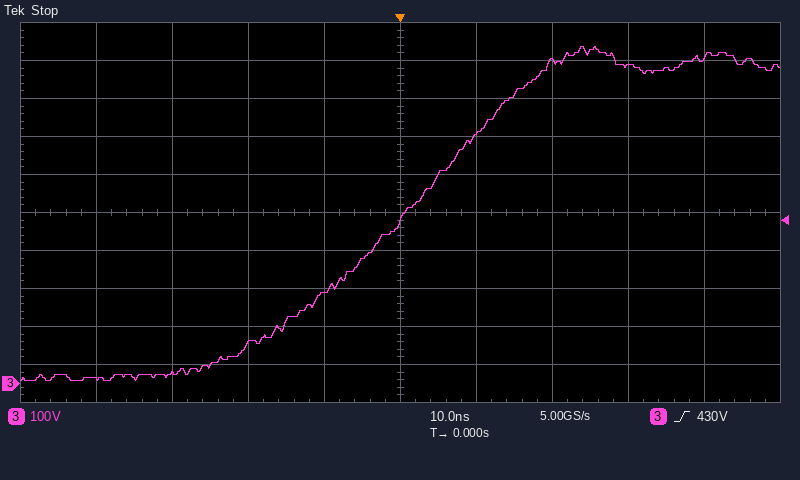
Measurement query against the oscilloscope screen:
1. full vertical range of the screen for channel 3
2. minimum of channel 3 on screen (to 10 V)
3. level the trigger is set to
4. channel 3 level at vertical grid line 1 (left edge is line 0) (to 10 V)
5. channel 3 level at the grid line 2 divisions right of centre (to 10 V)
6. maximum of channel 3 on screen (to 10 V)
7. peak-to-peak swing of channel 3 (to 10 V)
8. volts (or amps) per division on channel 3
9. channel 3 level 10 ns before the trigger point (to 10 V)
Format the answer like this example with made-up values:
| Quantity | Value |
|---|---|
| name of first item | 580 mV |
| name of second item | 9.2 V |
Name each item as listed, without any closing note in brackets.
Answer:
| Quantity | Value |
|---|---|
| full vertical range of the screen for channel 3 | 1 kV |
| minimum of channel 3 on screen | 10 V |
| level the trigger is set to | 430 V |
| channel 3 level at vertical grid line 1 (left edge is line 0) | 10 V |
| channel 3 level at the grid line 2 divisions right of centre | 850 V |
| maximum of channel 3 on screen | 890 V |
| peak-to-peak swing of channel 3 | 880 V |
| volts (or amps) per division on channel 3 | 100 V |
| channel 3 level 10 ns before the trigger point | 240 V |
